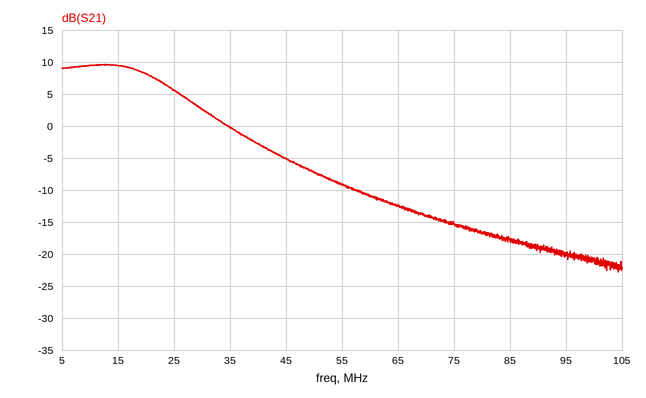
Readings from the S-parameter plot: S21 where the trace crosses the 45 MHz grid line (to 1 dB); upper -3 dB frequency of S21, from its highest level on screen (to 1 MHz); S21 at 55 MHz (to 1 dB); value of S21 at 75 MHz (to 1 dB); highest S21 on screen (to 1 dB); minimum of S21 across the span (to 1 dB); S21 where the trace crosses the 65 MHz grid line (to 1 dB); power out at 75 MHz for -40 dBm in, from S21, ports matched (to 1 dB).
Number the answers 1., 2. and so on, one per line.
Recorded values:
1. -5 dB
2. 23 MHz
3. -9 dB
4. -15 dB
5. 10 dB
6. -23 dB
7. -12 dB
8. -55 dBm
